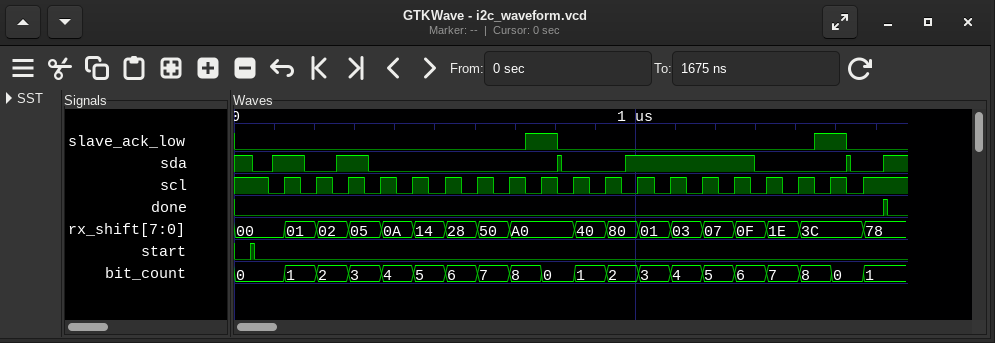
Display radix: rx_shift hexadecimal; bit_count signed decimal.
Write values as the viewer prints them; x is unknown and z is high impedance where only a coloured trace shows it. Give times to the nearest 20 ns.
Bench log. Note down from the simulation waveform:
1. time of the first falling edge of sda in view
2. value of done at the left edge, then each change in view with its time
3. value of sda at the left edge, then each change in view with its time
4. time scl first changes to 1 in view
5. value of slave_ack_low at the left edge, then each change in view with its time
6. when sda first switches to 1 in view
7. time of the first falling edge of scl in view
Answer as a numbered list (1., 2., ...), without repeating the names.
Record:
1. 40 ns
2. 0, 1 at 1620 ns, 0 at 1620 ns
3. 1, 0 at 40 ns, 1 at 100 ns, 0 at 180 ns, 1 at 260 ns, 0 at 340 ns, 1 at 800 ns, 0 at 820 ns, 1 at 980 ns, 0 at 1300 ns, 1 at 1520 ns, 0 at 1540 ns, 1 at 1620 ns
4. 120 ns
5. 0, 1 at 720 ns, 0 at 800 ns, 1 at 1440 ns, 0 at 1520 ns
6. 100 ns
7. 80 ns
